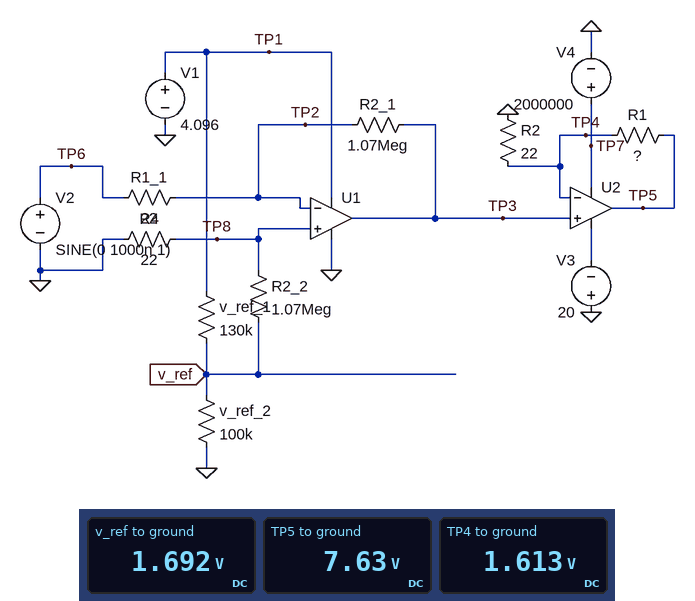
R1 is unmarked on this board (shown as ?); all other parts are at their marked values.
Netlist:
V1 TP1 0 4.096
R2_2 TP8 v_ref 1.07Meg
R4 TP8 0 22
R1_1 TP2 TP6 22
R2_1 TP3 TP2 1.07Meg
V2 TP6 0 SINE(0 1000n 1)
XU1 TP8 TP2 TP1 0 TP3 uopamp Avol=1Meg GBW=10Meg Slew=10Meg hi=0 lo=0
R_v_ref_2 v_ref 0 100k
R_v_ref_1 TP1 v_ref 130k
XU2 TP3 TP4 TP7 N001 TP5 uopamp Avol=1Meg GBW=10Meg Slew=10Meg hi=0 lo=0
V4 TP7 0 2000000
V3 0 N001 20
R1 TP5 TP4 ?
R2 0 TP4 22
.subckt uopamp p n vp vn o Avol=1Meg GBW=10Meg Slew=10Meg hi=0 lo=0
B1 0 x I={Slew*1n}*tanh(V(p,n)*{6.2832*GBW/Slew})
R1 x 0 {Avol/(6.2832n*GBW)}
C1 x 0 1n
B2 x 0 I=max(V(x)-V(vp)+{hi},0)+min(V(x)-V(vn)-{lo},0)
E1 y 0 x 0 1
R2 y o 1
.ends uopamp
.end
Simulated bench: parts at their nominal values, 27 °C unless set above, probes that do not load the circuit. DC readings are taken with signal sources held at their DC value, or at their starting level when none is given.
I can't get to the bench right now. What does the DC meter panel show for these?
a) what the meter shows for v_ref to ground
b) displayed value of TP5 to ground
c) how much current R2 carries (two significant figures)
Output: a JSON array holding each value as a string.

["1.692 V", "7.63 V", "73 mA"]
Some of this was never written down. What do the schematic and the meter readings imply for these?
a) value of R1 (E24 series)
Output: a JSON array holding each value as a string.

["82 Ω"]
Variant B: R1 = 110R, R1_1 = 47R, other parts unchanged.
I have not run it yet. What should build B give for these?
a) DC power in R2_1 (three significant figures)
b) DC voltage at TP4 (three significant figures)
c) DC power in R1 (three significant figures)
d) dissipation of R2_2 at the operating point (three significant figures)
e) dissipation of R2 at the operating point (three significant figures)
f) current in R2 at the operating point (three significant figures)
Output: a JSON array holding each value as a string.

["560 nW", "774 mV", "136 mW", "2.67 µW", "27.2 mW", "35.2 mA"]
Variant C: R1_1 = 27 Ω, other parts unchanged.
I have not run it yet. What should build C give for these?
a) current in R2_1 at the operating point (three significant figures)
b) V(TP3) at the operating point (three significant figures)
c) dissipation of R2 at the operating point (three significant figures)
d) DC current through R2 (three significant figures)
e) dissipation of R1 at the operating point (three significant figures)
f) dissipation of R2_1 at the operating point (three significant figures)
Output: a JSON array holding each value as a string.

["1.24 µA", "1.33 V", "79.9 mW", "60.3 mA", "298 mW", "1.64 µW"]
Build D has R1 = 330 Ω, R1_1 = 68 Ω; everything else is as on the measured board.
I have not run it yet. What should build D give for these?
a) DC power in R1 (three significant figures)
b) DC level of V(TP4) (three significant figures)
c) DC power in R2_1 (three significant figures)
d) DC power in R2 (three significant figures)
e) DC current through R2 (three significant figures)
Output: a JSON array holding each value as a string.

["198 mW", "539 mV", "271 nW", "13.2 mW", "24.5 mA"]
